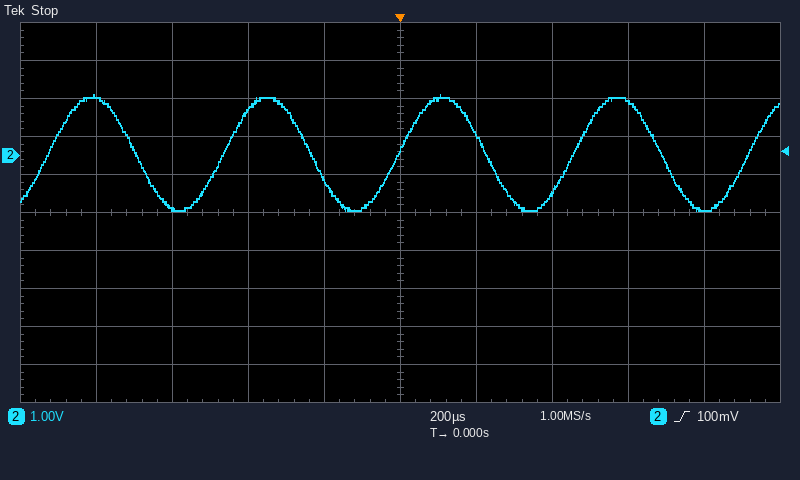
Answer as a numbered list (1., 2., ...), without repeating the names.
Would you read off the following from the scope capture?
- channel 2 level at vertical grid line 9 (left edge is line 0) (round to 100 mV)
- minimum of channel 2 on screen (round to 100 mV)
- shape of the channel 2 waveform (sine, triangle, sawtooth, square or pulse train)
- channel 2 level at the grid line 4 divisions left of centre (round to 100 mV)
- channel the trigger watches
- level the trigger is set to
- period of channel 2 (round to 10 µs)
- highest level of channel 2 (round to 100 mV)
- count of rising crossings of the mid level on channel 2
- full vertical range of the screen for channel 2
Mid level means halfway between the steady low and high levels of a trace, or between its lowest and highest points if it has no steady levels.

1. -1.4 V
2. -1.4 V
3. sine
4. 1.5 V
5. channel 2
6. 100 mV
7. 460 µs
8. 1.6 V
9. 5
10. 10 V
